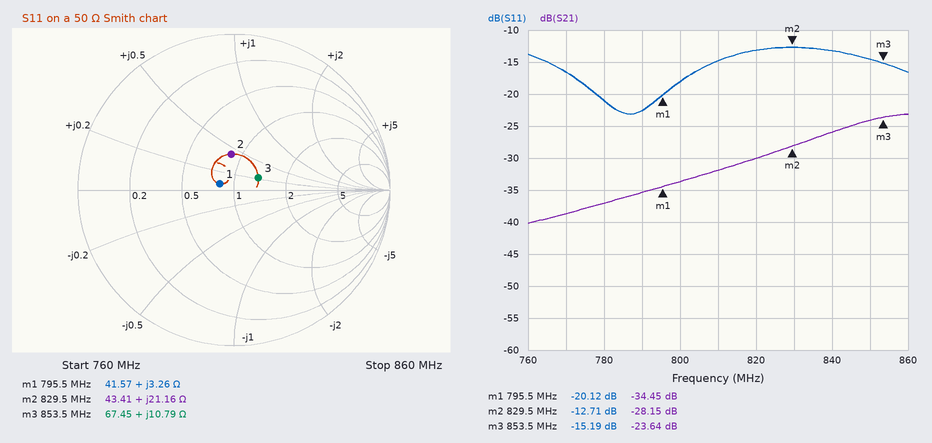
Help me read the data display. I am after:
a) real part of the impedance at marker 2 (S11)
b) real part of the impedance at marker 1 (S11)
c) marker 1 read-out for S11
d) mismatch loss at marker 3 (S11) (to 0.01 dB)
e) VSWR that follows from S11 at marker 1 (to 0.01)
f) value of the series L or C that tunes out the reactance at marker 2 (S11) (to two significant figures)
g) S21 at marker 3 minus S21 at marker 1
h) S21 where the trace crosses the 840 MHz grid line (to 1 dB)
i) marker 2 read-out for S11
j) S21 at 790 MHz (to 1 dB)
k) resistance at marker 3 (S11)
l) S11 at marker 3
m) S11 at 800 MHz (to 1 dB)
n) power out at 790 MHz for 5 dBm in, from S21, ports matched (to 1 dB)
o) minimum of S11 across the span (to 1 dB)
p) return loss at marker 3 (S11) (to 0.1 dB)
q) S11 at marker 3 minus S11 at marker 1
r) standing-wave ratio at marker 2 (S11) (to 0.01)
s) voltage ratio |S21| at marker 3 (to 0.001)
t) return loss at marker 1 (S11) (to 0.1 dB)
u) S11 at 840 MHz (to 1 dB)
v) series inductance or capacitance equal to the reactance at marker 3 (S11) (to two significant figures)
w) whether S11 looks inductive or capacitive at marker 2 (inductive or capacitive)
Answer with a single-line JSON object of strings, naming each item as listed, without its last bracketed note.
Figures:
{"real part of the impedance at marker 2": "43.41 Ω", "real part of the impedance at marker 1": "41.57 Ω", "marker 1 read-out for S11": "-20.12 dB", "mismatch loss at marker 3 (S11)": "0.13 dB", "VSWR that follows from S11 at marker 1": "1.22", "value of the series L or C that tunes out the reactance at marker 2 (S11)": "9.1 pF", "S21 at marker 3 minus S21 at marker 1": "10.81 dB", "S21 where the trace crosses the 840 MHz grid line": "-26 dB", "marker 2 read-out for S11": "-12.71 dB", "S21 at 790 MHz": "-35 dB", "resistance at marker 3": "67.45 Ω", "S11 at marker 3": "-15.19 dB", "S11 at 800 MHz": "-18 dB", "power out at 790 MHz for 5 dBm in, from S21, ports matched": "-30 dBm", "minimum of S11 across the span": "-23 dB", "return loss at marker 3 (S11)": "15.2 dB", "S11 at marker 3 minus S11 at marker 1": "4.93 dB", "standing-wave ratio at marker 2 (S11)": "1.60", "voltage ratio |S21| at marker 3": "0.066", "return loss at marker 1 (S11)": "20.1 dB", "S11 at 840 MHz": "-13 dB", "series inductance or capacitance equal to the reactance at marker 3 (S11)": "2.0 nH", "whether S11 looks inductive or capacitive at marker 2": "inductive"}
